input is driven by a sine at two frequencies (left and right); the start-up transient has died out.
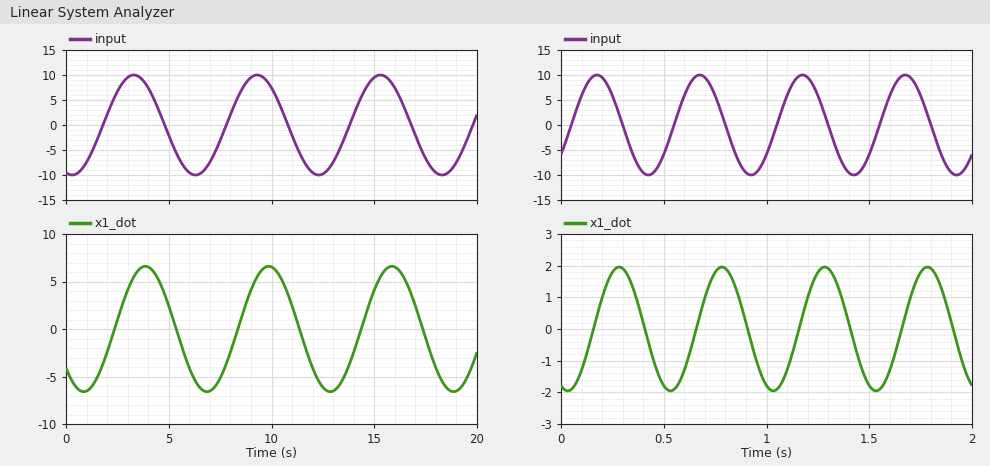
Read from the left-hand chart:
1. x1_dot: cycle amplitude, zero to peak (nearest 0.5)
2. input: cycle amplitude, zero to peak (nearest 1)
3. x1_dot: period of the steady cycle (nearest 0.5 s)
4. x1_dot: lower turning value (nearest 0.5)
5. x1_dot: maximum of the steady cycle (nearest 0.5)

6.5
10
6.0 s
-6.5
6.5
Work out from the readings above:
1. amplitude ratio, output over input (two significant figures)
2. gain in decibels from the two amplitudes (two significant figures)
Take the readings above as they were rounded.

0.65
-3.7 dB
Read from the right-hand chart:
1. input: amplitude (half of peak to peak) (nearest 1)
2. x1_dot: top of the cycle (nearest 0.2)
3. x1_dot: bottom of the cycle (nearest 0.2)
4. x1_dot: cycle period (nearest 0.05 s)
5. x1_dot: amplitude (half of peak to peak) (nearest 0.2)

10
2.0
-2.0
0.50 s
2.0
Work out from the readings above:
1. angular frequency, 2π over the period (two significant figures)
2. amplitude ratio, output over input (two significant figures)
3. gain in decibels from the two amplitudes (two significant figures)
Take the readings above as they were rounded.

13 rad/s
0.20
-14 dB
